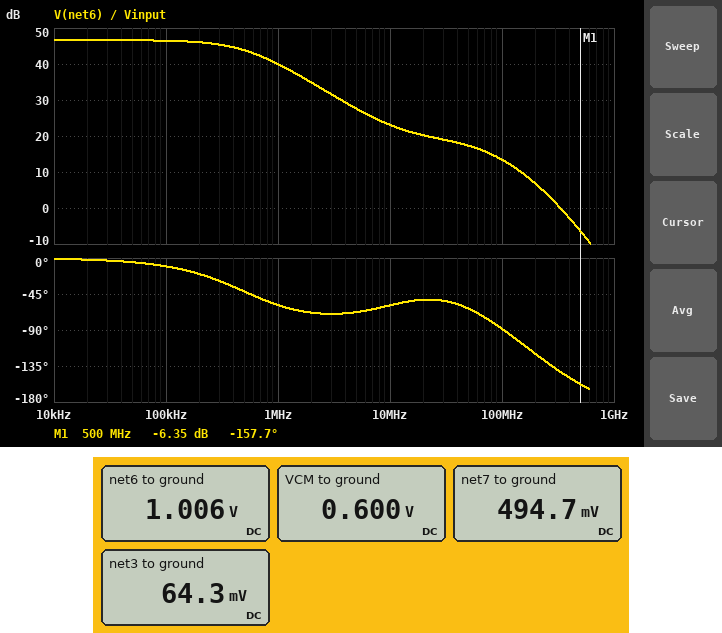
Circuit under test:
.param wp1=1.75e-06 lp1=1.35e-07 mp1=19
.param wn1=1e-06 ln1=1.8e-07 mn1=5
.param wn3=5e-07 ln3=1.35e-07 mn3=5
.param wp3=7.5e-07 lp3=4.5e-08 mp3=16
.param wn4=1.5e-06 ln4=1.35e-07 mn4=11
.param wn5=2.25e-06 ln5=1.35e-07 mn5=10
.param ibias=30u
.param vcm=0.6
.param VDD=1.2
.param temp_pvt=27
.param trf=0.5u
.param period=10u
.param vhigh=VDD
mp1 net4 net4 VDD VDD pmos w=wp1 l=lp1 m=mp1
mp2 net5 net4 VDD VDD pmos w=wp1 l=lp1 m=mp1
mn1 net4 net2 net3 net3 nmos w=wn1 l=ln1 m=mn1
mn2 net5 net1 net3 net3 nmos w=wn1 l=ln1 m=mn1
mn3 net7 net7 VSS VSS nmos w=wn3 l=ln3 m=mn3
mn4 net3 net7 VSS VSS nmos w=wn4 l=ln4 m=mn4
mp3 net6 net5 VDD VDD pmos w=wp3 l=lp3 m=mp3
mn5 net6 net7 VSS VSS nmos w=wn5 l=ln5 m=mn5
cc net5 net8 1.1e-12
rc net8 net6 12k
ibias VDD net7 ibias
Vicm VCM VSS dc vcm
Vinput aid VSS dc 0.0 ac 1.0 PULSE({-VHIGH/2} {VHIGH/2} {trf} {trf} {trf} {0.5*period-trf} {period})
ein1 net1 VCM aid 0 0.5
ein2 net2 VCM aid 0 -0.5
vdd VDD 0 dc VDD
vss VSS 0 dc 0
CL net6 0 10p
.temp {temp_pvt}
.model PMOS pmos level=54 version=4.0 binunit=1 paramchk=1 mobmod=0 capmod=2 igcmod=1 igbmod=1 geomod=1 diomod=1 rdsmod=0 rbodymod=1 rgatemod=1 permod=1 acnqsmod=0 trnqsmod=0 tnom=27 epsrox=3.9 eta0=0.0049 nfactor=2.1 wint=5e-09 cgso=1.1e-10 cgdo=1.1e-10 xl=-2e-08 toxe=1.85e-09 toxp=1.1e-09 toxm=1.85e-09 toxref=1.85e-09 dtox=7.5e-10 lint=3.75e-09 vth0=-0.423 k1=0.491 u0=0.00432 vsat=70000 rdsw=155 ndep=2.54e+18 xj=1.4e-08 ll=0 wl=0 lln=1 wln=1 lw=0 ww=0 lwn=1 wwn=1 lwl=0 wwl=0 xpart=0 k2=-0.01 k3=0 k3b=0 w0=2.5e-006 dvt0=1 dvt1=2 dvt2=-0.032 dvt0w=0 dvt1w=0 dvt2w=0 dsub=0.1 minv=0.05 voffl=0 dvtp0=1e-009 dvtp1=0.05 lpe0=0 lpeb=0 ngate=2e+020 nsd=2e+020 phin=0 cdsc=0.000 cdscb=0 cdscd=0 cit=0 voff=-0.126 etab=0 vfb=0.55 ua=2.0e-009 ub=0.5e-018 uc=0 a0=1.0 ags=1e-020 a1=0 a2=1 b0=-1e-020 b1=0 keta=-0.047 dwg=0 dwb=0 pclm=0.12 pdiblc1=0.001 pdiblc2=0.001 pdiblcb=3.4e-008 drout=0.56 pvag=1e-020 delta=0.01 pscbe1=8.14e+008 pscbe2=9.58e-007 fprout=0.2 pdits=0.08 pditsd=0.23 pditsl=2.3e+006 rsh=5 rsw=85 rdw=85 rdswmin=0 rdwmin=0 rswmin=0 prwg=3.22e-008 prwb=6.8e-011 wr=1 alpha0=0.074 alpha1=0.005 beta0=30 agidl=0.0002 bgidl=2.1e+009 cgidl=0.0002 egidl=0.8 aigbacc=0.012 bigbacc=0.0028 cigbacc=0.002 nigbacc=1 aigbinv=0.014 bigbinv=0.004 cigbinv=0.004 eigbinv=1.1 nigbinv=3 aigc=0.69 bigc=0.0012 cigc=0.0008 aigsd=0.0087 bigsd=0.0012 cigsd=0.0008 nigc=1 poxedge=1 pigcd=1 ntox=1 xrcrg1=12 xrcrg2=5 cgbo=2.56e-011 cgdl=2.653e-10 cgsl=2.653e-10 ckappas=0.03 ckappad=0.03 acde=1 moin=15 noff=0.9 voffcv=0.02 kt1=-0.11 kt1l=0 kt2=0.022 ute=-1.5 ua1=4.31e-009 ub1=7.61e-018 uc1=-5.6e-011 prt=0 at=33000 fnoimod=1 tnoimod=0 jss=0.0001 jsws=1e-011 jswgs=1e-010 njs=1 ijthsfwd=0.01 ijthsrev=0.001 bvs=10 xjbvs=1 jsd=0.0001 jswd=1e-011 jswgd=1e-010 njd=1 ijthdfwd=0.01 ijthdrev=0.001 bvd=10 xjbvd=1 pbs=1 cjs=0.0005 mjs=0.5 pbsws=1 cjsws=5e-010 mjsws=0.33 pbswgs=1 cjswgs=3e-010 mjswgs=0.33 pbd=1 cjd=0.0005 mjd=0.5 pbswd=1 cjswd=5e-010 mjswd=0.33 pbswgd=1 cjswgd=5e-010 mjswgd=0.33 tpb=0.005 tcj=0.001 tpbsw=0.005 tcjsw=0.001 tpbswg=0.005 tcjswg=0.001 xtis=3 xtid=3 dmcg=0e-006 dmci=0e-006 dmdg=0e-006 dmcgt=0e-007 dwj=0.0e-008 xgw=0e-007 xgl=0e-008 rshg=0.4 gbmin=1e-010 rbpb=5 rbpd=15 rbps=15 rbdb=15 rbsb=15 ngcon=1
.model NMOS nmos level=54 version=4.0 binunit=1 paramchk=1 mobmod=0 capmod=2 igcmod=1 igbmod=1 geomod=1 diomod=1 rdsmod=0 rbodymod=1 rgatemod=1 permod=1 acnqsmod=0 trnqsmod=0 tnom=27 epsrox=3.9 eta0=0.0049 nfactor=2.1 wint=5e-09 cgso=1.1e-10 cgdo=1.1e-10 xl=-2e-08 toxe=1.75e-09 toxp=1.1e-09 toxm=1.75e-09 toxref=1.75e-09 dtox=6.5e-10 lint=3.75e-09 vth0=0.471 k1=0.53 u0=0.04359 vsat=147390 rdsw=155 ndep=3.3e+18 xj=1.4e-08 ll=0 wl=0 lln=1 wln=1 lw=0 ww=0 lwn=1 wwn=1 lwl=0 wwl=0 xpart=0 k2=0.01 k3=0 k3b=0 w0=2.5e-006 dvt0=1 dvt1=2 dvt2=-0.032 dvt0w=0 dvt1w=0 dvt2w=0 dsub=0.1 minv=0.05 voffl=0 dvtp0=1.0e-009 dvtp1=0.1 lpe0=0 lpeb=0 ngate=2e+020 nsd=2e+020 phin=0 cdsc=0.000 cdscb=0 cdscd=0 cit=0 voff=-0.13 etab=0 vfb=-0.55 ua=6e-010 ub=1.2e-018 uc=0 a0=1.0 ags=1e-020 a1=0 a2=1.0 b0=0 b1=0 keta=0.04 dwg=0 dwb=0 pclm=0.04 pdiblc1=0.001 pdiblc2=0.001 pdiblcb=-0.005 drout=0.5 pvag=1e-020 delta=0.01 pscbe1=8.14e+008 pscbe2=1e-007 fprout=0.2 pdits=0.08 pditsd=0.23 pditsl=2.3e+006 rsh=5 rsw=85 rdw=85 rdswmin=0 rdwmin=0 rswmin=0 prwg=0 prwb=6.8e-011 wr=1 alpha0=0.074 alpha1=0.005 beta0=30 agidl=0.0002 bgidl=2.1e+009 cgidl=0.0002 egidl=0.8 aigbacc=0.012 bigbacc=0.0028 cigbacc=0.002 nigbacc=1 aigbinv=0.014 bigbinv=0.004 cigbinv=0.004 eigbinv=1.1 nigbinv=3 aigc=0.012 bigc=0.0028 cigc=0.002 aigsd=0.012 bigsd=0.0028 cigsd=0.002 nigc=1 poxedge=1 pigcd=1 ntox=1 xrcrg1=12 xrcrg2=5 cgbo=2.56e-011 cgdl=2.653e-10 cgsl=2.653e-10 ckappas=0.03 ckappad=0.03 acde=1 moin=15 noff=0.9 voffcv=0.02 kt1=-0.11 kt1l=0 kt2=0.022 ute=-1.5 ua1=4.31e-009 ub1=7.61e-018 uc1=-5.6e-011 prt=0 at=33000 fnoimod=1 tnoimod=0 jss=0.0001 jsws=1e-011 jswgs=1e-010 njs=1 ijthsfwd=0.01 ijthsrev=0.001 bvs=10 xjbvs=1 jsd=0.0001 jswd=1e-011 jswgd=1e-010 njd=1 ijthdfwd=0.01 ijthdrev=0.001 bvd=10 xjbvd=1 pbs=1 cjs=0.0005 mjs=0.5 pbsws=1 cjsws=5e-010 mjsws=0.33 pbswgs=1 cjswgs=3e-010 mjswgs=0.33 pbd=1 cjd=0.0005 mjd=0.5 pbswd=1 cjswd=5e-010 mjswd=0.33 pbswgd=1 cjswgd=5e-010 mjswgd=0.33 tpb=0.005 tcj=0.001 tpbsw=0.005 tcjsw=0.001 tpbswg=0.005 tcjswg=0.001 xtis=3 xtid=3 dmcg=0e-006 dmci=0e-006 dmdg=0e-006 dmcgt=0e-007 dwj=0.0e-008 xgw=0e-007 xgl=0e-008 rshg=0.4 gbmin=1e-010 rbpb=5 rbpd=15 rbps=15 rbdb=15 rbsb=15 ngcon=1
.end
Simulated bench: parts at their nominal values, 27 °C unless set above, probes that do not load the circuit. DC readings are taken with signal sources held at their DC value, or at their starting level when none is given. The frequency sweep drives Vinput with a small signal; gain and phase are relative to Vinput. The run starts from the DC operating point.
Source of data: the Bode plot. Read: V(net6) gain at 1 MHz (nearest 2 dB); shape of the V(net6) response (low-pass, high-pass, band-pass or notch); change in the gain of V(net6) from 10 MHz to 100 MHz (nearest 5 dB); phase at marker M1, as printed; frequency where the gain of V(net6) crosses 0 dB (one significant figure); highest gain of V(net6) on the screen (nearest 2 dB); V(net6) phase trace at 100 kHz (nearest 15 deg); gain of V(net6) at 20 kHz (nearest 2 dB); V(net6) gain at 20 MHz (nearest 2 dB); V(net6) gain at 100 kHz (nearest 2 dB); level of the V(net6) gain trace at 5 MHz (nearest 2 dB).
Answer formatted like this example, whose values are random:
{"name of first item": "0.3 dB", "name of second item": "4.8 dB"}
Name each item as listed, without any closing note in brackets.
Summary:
{"V(net6) gain at 1 MHz": "40 dB", "shape of the V(net6) response": "low-pass", "change in the gain of V(net6) from 10 MHz to 100 MHz": "-10 dB", "phase at marker M1, as printed": "-157.7 deg", "frequency where the gain of V(net6) crosses 0 dB": "300 MHz", "highest gain of V(net6) on the screen": "46 dB", "V(net6) phase trace at 100 kHz": "-15 deg", "gain of V(net6) at 20 kHz": "46 dB", "V(net6) gain at 20 MHz": "20 dB", "V(net6) gain at 100 kHz": "46 dB", "level of the V(net6) gain trace at 5 MHz": "28 dB"}
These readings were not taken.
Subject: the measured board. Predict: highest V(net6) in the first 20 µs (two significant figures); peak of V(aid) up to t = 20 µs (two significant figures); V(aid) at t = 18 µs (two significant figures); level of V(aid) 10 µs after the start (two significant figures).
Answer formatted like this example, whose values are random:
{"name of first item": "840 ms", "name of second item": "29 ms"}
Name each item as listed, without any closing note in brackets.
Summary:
{"highest V(net6) in the first 20 µs": "1.2 V", "peak of V(aid) up to t = 20 µs": "600 mV", "V(aid) at t = 18 µs": "-600 mV", "level of V(aid) 10 µs after the start": "-600 mV"}
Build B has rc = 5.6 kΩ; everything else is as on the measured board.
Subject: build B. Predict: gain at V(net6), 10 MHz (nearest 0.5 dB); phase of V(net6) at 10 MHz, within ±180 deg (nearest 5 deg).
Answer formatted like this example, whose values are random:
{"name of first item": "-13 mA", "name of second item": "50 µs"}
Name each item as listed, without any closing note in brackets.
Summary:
{"gain at V(net6), 10 MHz": "21.5 dB", "phase of V(net6) at 10 MHz, within ±180 deg": "-75 deg"}
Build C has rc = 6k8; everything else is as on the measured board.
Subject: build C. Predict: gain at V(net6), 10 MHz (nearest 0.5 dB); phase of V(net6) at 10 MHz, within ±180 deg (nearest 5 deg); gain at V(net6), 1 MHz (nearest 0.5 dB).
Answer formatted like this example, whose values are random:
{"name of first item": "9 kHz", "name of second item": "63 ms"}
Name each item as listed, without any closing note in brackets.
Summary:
{"gain at V(net6), 10 MHz": "22.0 dB", "phase of V(net6) at 10 MHz, within ±180 deg": "-75 deg", "gain at V(net6), 1 MHz": "40.0 dB"}
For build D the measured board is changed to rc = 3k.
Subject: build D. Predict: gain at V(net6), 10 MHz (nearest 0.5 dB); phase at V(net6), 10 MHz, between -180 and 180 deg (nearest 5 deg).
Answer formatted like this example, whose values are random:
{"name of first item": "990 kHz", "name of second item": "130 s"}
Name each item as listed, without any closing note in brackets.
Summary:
{"gain at V(net6), 10 MHz": "21.5 dB", "phase at V(net6), 10 MHz, between -180 and 180 deg": "-85 deg"}
